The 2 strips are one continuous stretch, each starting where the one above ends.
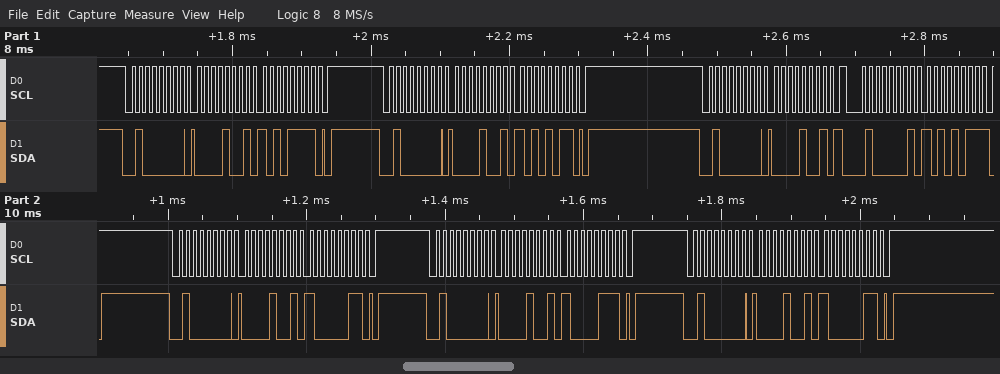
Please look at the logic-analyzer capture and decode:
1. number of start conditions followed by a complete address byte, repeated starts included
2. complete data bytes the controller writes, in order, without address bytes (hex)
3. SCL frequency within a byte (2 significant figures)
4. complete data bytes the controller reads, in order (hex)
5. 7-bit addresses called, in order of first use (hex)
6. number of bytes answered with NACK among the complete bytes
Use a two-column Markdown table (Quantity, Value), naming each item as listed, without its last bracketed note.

| Quantity | Value |
|---|---|
| number of start conditions followed by a complete address byte, repeated starts included | 7 |
| complete data bytes the controller writes, in order, without address bytes | 09 AF 09 AB 09 09 83 09 87 09 83 |
| SCL frequency within a byte | 100 kHz |
| complete data bytes the controller reads, in order | AB |
| 7-bit addresses called, in order of first use | 0x20 |
| number of bytes answered with NACK among the complete bytes | 1 |
